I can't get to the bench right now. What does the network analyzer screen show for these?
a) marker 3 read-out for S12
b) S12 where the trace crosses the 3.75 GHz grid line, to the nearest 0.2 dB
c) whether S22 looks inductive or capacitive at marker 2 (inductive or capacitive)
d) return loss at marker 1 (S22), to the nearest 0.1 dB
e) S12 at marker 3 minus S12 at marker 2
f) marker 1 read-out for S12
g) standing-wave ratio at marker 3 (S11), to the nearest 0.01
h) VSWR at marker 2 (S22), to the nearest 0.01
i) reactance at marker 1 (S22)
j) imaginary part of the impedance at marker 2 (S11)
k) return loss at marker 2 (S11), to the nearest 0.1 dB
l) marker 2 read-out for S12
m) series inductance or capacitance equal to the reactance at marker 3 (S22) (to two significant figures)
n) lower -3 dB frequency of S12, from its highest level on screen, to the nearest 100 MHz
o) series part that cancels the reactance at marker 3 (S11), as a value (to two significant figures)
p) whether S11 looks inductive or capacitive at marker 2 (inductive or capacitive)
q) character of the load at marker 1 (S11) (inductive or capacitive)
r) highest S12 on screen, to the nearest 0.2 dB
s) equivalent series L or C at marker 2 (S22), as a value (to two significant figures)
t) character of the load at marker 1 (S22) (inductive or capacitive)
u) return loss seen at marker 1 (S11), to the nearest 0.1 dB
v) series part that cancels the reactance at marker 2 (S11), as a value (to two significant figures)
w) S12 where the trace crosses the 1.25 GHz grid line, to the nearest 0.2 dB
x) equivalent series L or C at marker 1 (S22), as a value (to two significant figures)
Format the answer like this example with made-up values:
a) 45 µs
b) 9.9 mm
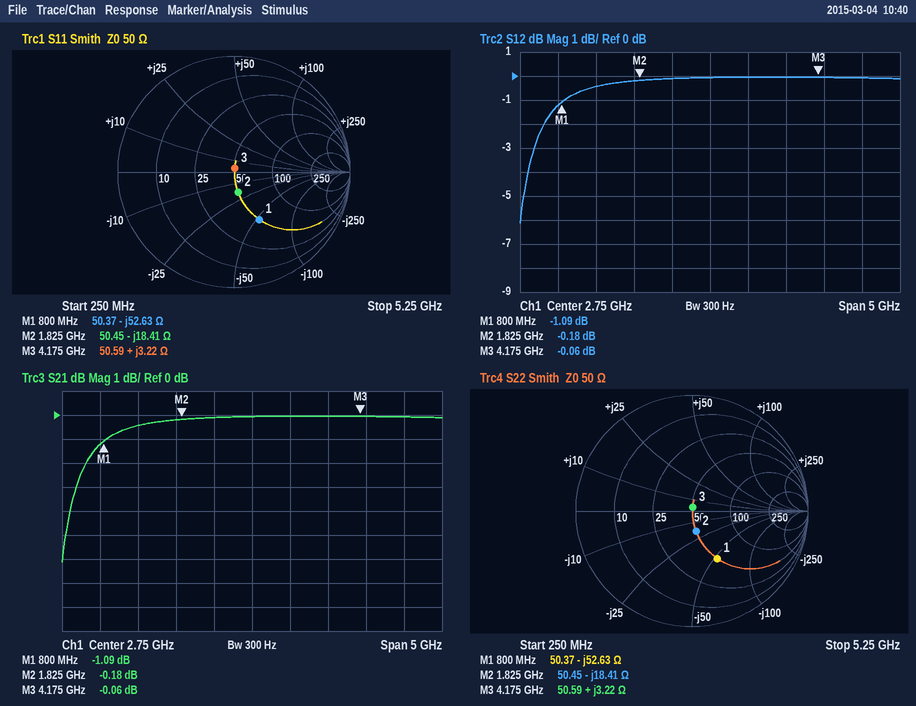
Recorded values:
a) -0.06 dB
b) 0.0 dB
c) capacitive
d) 6.7 dB
e) 0.12 dB
f) -1.09 dB
g) 1.07
h) 1.44
i) -52.63 Ω
j) -18.41 Ω
k) 14.9 dB
l) -0.18 dB
m) 120 pH
n) 400 MHz
o) 12 pF
p) capacitive
q) capacitive
r) 0.0 dB
s) 4.7 pF
t) capacitive
u) 6.7 dB
v) 1.6 nH
w) -0.4 dB
x) 3.8 pF
